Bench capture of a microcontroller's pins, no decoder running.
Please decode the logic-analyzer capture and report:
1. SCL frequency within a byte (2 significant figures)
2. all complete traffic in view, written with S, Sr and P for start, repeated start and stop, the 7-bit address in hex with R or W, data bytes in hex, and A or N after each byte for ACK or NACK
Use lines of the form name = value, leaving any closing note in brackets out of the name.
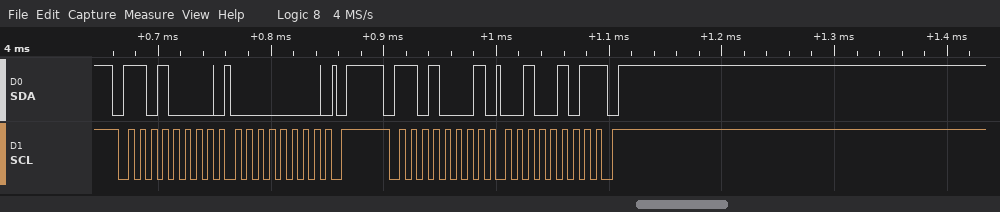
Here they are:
SCL frequency within a byte = 100 kHz
all complete traffic in view, written with S, Sr and P for start, repeated start and stop, the 7-bit address in hex with R or W, data bytes in hex, and A or N after each byte for ACK or NACK = S 68W A 00 A P S 68R A 25 N P
